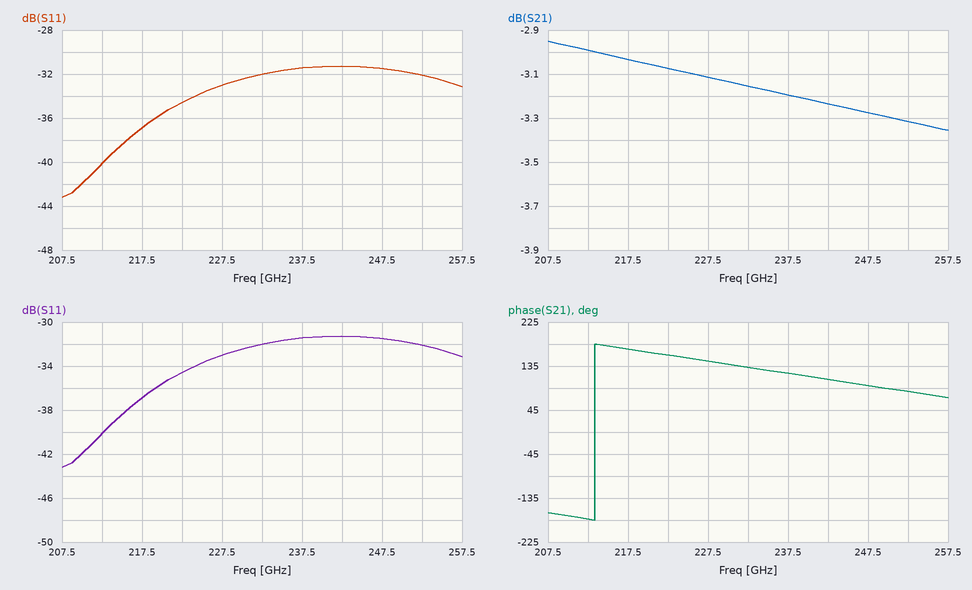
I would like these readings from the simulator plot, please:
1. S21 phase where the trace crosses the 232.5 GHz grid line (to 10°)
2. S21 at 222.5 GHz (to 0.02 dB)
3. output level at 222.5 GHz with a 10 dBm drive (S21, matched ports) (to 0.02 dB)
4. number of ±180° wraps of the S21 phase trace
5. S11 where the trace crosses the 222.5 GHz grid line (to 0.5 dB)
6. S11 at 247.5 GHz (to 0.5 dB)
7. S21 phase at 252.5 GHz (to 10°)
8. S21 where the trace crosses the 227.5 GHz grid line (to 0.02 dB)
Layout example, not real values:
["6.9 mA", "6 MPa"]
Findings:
["130°", "-3.08 dB", "6.92 dBm", "1", "-34.5 dB", "-31.5 dB", "80°", "-3.12 dB"]
